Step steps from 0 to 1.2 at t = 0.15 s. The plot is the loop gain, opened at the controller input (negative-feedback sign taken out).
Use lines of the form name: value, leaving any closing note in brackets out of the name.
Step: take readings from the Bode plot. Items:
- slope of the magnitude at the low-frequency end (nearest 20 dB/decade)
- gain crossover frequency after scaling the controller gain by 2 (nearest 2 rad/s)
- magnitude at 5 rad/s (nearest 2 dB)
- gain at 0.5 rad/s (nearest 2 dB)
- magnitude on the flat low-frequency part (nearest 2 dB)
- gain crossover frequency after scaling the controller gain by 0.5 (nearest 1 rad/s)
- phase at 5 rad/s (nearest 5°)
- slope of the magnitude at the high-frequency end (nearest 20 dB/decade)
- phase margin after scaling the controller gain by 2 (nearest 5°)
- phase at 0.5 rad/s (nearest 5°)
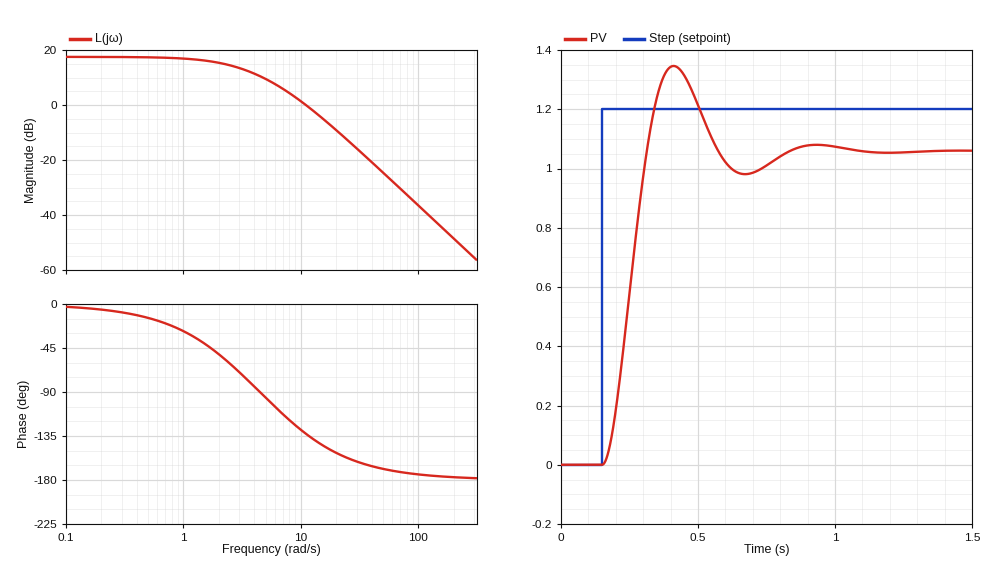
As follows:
slope of the magnitude at the low-frequency end: 0 dB/decade
gain crossover frequency after scaling the controller gain by 2: 16 rad/s
magnitude at 5 rad/s: 10 dB
gain at 0.5 rad/s: 18 dB
magnitude on the flat low-frequency part: 18 dB
gain crossover frequency after scaling the controller gain by 0.5: 7 rad/s
phase at 5 rad/s: -95°
slope of the magnitude at the high-frequency end: -40 dB/decade
phase margin after scaling the controller gain by 2: 35°
phase at 0.5 rad/s: -15°
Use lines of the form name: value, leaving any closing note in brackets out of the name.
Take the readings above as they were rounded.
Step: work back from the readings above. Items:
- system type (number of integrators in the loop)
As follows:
system type: 0
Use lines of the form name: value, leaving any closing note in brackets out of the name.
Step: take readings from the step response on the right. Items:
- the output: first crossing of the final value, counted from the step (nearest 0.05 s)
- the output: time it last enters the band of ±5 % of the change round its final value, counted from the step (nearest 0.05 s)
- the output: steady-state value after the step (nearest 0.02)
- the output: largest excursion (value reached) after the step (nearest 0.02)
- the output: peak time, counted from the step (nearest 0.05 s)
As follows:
the output: first crossing of the final value, counted from the step: 0.15 s
the output: time it last enters the band of ±5 % of the change round its final value, counted from the step: 0.60 s
the output: steady-state value after the step: 1.06
the output: largest excursion (value reached) after the step: 1.34
the output: peak time, counted from the step: 0.25 s
